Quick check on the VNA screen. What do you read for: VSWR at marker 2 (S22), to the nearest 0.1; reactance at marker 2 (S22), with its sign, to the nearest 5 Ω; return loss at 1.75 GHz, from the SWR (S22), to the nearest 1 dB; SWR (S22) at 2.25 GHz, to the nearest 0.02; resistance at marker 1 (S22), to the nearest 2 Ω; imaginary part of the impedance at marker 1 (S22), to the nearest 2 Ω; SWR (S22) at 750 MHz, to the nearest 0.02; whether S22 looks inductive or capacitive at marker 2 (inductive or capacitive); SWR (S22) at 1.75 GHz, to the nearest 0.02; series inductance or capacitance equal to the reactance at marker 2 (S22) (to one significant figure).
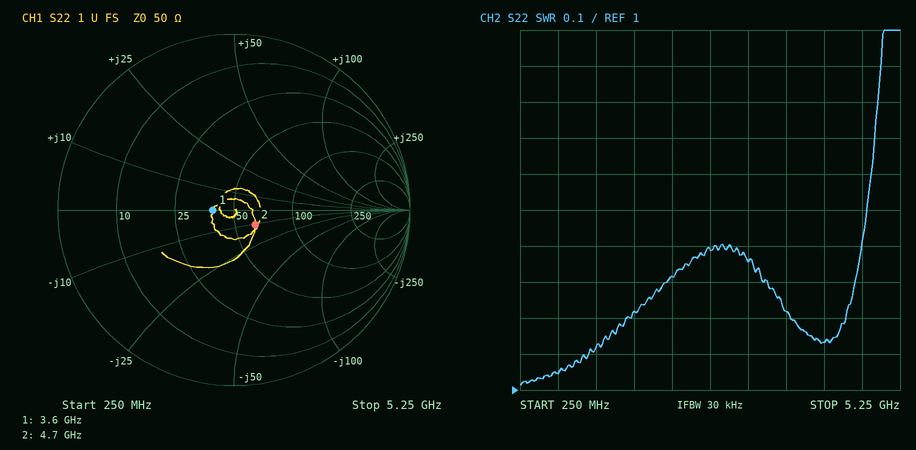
1.3
-10 Ω
20 dB
1.32
40 Ω
0 Ω
1.04
capacitive
1.22
3 pF
